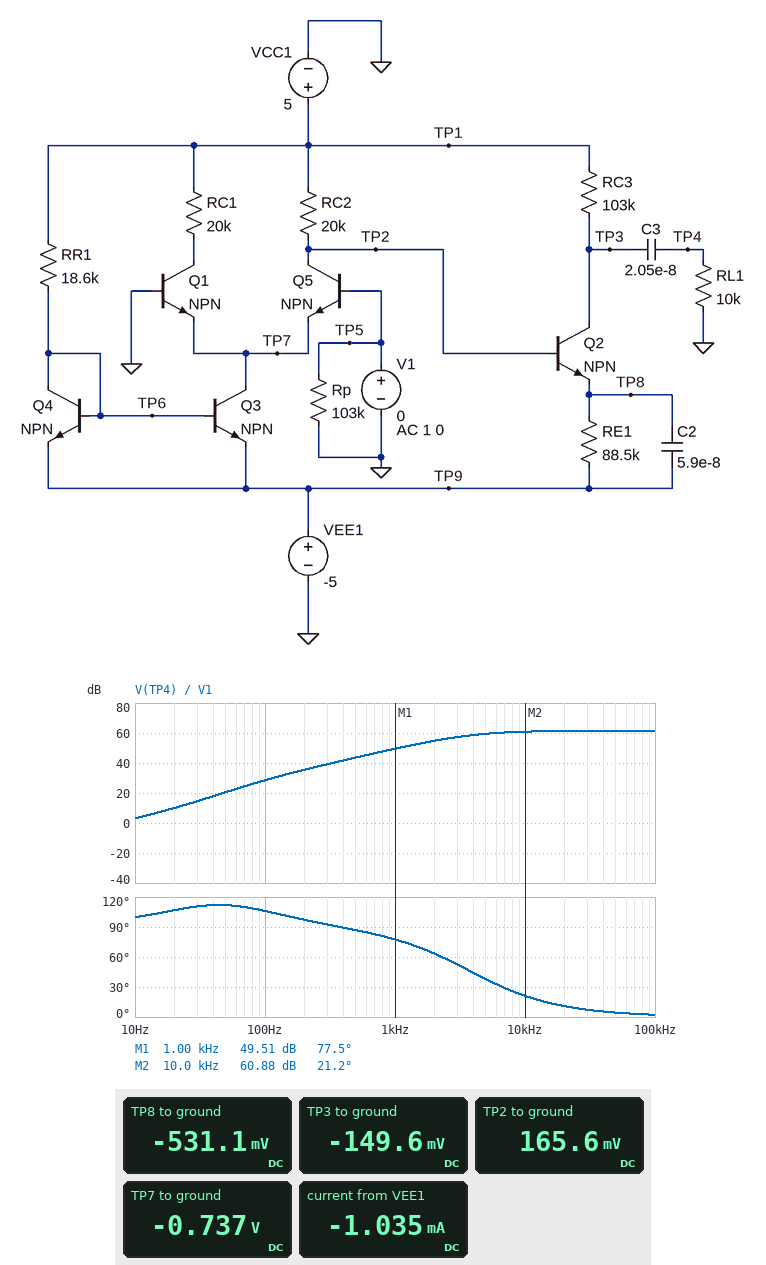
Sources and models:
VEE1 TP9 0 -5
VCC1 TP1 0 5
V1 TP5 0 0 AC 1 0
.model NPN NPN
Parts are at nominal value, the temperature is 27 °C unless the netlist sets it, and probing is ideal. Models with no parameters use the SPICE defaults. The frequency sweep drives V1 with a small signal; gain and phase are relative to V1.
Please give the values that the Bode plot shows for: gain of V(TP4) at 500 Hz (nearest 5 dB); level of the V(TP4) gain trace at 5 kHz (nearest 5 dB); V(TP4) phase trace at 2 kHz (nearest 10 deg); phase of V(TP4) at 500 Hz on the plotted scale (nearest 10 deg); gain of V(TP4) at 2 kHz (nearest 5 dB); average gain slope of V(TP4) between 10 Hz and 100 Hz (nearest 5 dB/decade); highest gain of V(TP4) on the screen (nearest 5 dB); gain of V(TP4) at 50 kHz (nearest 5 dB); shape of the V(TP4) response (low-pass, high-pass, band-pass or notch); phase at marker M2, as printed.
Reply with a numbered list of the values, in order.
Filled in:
1. 45 dB
2. 60 dB
3. 60 deg
4. 90 deg
5. 55 dB
6. 25 dB/decade
7. 60 dB
8. 60 dB
9. high-pass
10. 21.2 deg
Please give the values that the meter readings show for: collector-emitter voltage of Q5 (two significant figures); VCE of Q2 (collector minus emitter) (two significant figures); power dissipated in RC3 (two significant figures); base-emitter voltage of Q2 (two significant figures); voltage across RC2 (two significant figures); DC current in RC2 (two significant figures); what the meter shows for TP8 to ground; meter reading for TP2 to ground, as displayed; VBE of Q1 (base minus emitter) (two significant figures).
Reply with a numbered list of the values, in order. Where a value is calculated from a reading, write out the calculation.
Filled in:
1. 165.6 mV - (-737 mV) = 900 mV
2. -149.6 mV - (-531.1 mV) = 380 mV
3. (5 V - (-149.6 mV))^2 / 103 kΩ = 260 µW
4. 165.6 mV - (-531.1 mV) = 700 mV
5. 5 V - 165.6 mV = 4.8 V
6. (5 V - 165.6 mV) / 20 kΩ = 240 µA
7. -531.1 mV
8. 165.6 mV
9. 0 V - (-737 mV) = 740 mV
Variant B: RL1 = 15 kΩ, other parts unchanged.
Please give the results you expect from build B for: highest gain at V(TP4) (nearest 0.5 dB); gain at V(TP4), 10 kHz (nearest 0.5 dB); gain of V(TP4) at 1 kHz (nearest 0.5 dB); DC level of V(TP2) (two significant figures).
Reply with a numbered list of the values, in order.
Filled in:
1. 64.5 dB
2. 64.0 dB
3. 52.5 dB
4. 170 mV
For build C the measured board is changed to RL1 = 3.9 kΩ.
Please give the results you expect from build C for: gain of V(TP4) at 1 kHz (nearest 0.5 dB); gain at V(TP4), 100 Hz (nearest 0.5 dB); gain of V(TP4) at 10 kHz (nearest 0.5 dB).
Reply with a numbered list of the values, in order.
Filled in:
1. 42.0 dB
2. 20.5 dB
3. 53.0 dB
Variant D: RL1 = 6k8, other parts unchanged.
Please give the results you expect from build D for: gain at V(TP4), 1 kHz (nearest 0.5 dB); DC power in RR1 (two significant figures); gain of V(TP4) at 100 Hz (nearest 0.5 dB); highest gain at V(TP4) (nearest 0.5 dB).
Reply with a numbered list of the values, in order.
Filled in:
1. 46.5 dB
2. 4.6 mW
3. 25.5 dB
4. 58.5 dB
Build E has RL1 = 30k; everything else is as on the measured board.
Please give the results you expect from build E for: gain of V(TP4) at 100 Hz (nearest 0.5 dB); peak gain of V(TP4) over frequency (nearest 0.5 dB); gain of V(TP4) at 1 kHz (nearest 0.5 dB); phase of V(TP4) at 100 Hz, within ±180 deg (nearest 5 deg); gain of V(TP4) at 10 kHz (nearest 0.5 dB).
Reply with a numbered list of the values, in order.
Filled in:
1. 37.0 dB
2. 69.5 dB
3. 57.5 dB
4. 100 deg
5. 69.0 dB
